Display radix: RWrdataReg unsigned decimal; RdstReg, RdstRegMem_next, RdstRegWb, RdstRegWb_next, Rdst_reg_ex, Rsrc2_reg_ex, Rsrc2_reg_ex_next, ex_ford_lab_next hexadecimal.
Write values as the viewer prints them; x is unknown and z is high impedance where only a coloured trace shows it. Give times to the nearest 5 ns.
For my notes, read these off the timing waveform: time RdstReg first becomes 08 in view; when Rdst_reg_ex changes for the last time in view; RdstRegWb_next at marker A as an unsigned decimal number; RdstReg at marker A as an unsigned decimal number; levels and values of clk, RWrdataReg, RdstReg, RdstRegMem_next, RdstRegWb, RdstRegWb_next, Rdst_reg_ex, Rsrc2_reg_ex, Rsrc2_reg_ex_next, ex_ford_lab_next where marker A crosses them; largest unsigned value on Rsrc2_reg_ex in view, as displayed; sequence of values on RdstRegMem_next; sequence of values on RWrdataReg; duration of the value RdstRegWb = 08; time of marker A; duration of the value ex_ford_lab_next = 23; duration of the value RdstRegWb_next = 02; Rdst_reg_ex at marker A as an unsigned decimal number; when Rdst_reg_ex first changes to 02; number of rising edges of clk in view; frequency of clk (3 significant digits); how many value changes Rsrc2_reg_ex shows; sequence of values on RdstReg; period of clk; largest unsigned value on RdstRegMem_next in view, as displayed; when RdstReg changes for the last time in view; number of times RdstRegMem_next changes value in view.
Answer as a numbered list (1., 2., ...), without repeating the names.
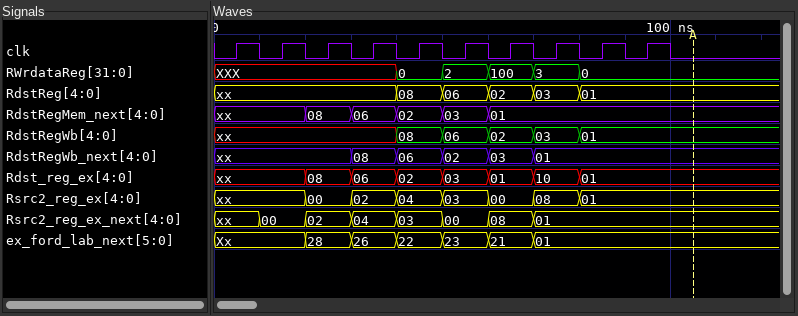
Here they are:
1. 40 ns
2. 80 ns
3. 1
4. 1
5. clk=0, RWrdataReg=0, RdstReg=01, RdstRegMem_next=01, RdstRegWb=01, RdstRegWb_next=01, Rdst_reg_ex=01, Rsrc2_reg_ex=01, Rsrc2_reg_ex_next=01, ex_ford_lab_next=01
6. 08
7. xx, 08, 06, 02, 03, 01
8. XXX, 0, 2, 100, 3, 0
9. 10 ns
10. 105 ns
11. 10 ns
12. 10 ns
13. 1
14. 40 ns
15. 10
16. 100 MHz
17. 7
18. xx, 08, 06, 02, 03, 01
19. 10 ns
20. 08
21. 80 ns
22. 5
